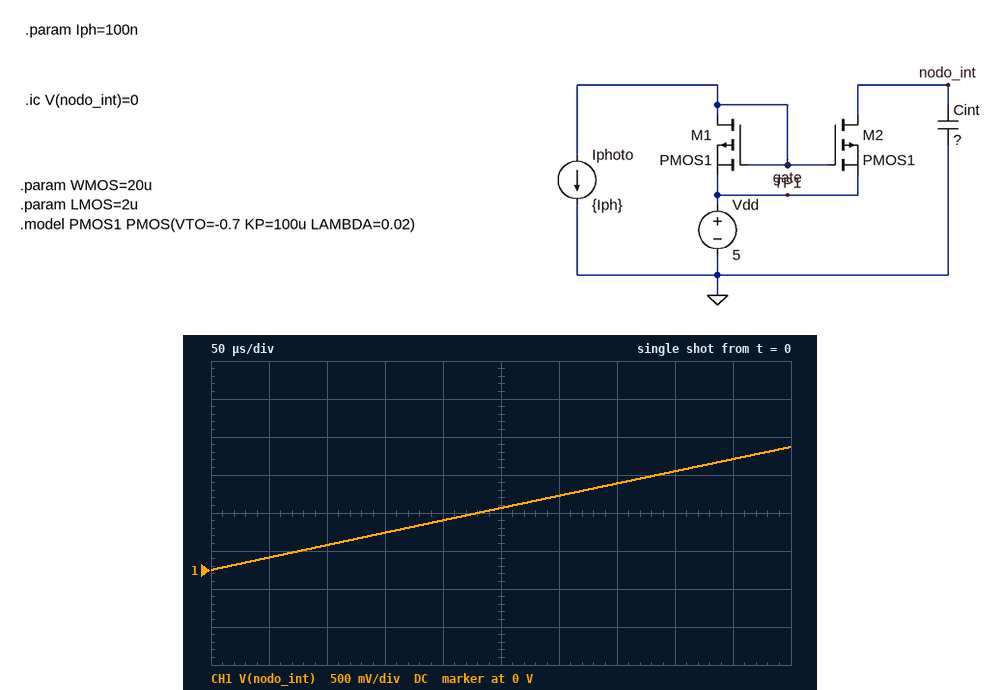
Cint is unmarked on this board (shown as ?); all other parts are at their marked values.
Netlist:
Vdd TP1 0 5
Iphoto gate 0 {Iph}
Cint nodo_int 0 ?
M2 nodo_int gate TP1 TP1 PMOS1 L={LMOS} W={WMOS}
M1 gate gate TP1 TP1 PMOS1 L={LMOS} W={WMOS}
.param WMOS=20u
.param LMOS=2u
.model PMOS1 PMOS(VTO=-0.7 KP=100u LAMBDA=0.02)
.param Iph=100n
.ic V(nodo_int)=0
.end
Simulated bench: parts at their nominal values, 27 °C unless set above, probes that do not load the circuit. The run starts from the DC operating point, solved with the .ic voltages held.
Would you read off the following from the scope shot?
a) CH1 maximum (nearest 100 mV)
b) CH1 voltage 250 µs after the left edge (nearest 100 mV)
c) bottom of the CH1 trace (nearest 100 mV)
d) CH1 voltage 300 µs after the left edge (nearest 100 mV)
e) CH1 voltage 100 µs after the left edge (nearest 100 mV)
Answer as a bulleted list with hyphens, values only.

- 1.6 V
- 800 mV
- 0 V
- 1.0 V
- 300 mV
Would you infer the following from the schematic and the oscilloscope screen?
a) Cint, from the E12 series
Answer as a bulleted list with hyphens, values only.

- 33 pF
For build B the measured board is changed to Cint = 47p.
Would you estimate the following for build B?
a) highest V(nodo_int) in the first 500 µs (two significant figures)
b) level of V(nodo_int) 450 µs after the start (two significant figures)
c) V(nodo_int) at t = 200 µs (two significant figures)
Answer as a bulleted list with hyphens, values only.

- 1.1 V
- 1.0 V
- 460 mV
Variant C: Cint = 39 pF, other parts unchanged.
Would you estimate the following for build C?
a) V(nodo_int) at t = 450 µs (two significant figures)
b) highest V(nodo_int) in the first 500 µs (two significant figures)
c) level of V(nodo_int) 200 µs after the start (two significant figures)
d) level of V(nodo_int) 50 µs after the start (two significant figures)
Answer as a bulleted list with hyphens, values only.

- 1.2 V
- 1.4 V
- 550 mV
- 140 mV
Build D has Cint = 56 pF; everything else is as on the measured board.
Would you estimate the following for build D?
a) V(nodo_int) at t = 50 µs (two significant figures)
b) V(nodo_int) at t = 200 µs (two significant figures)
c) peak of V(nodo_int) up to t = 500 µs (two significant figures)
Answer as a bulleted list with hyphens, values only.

- 97 mV
- 390 mV
- 960 mV
